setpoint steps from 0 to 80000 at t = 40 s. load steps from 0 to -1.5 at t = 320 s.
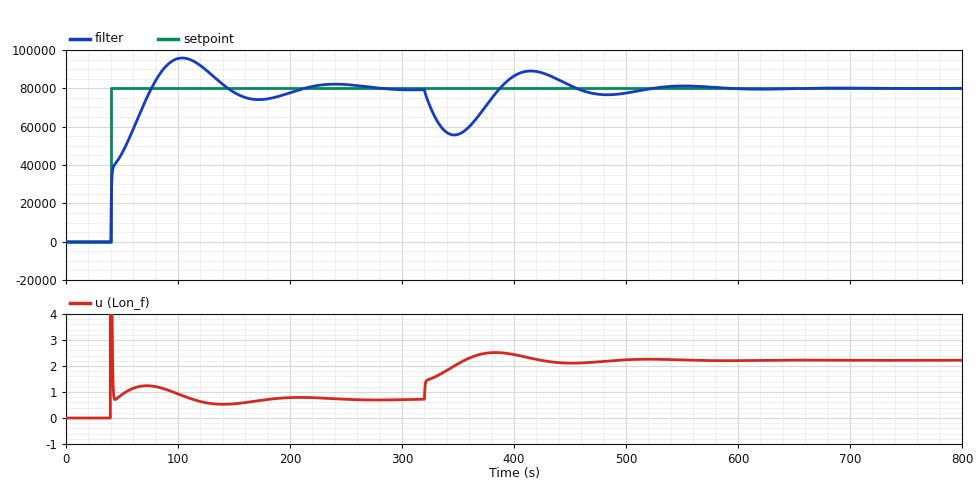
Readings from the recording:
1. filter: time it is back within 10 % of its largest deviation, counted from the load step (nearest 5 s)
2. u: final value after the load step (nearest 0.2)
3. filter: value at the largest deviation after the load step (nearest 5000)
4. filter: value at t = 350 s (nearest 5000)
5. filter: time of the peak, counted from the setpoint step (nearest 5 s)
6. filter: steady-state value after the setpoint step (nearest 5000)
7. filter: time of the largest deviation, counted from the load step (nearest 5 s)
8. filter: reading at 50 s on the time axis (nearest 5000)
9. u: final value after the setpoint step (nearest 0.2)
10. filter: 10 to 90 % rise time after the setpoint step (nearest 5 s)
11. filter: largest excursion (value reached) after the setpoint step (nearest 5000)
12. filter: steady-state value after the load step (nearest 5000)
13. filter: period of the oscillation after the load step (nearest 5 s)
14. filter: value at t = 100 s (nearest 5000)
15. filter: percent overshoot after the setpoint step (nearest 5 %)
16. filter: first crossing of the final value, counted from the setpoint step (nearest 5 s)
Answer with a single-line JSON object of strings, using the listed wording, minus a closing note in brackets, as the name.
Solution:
{"filter: time it is back within 10 % of its largest deviation, counted from the load step": "180 s", "u: final value after the load step": "2.2", "filter: value at the largest deviation after the load step": "55000", "filter: value at t = 350 s": "55000", "filter: time of the peak, counted from the setpoint step": "65 s", "filter: steady-state value after the setpoint step": "80000", "filter: time of the largest deviation, counted from the load step": "25 s", "filter: reading at 50 s on the time axis": "45000", "u: final value after the setpoint step": "0.8", "filter: 10 to 90 % rise time after the setpoint step": "30 s", "filter: largest excursion (value reached) after the setpoint step": "95000", "filter: steady-state value after the load step": "80000", "filter: period of the oscillation after the load step": "135 s", "filter: value at t = 100 s": "95000", "filter: percent overshoot after the setpoint step": "20 %", "filter: first crossing of the final value, counted from the setpoint step": "35 s"}
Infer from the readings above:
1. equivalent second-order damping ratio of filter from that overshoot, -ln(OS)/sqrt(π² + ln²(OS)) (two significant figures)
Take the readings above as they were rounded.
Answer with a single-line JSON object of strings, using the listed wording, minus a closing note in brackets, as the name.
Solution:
{"equivalent second-order damping ratio of filter from that overshoot, -ln(OS)/sqrt(π² + ln²(OS))": "0.46"}
